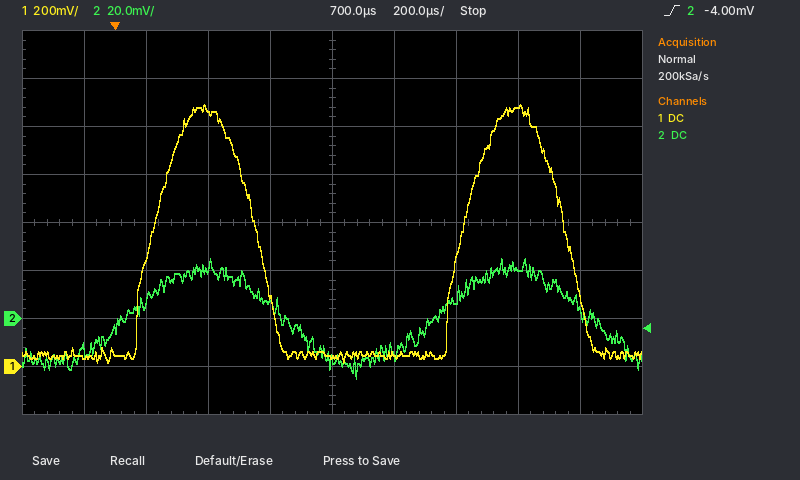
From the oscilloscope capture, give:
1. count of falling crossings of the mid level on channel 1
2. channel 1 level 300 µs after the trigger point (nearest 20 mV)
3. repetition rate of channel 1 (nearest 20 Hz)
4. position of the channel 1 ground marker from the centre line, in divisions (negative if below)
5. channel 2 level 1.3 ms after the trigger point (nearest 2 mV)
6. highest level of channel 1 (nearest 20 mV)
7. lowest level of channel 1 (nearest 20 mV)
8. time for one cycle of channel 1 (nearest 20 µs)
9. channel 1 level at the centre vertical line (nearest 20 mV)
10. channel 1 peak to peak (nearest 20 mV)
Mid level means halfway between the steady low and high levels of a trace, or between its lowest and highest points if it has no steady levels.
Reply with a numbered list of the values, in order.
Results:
1. 2
2. 1.06 V
3. 1.00 kHz
4. -3.0 div
5. 20 mV
6. 1.10 V
7. 20 mV
8. 1.00 ms
9. 40 mV
10. 1.08 V
